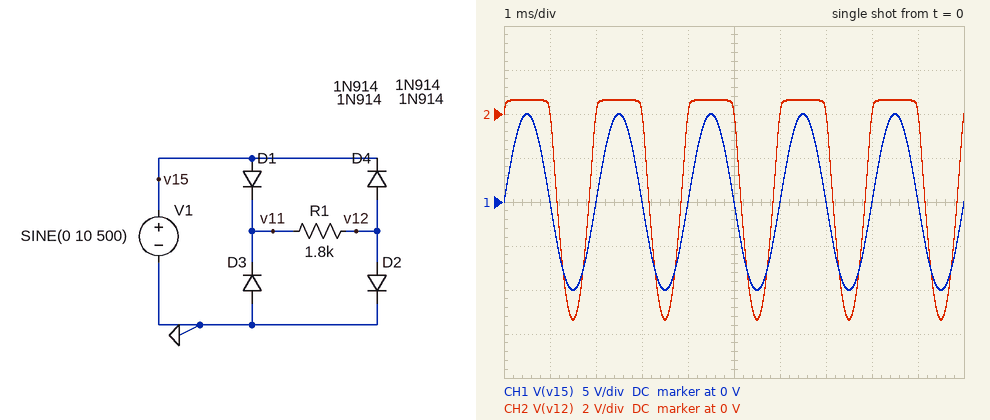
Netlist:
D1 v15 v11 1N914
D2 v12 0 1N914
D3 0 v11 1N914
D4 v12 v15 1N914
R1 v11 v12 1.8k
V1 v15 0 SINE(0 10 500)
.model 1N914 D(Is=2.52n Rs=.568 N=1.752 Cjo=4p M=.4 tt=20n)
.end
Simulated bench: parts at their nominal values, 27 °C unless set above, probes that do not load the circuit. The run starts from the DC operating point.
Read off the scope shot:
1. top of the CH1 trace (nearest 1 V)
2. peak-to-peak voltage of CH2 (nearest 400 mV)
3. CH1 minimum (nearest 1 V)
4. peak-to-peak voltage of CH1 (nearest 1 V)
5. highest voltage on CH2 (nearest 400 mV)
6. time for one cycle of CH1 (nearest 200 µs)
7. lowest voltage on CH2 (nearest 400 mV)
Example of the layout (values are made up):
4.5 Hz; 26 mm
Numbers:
10 V; 10.0 V; -10 V; 20 V; 800 mV; 2.0 ms; -9.2 V
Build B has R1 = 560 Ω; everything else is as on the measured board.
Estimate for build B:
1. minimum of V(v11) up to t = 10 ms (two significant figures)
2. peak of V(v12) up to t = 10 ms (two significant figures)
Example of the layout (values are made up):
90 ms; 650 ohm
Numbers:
-720 mV; 720 mV
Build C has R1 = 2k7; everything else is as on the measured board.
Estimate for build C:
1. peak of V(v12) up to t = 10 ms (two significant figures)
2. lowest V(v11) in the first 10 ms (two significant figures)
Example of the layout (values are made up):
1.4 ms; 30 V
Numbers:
640 mV; -640 mV
